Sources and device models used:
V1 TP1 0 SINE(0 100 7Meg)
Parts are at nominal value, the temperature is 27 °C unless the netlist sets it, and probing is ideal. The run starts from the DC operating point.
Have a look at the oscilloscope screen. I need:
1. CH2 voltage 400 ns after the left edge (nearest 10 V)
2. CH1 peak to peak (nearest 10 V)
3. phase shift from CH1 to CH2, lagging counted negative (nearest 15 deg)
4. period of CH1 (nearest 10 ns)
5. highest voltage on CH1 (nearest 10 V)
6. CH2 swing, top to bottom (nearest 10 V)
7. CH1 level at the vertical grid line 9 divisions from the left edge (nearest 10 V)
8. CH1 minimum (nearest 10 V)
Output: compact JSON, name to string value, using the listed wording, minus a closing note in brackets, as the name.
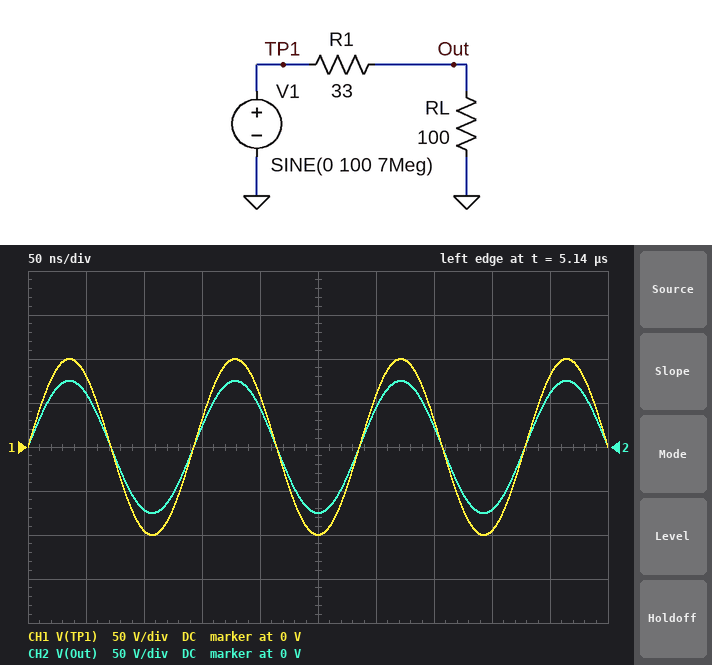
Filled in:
{"CH2 voltage 400 ns after the left edge": "-70 V", "CH1 peak to peak": "200 V", "phase shift from CH1 to CH2, lagging counted negative": "0 deg", "period of CH1": "140 ns", "highest voltage on CH1": "100 V", "CH2 swing, top to bottom": "150 V", "CH1 level at the vertical grid line 9 divisions from the left edge": "80 V", "CH1 minimum": "-100 V"}
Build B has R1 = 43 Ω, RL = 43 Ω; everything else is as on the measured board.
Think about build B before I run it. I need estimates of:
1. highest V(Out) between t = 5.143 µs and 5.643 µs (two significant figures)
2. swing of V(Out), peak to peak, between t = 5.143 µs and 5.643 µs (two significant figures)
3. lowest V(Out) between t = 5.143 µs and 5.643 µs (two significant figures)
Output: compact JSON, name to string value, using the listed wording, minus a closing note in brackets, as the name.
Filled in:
{"highest V(Out) between t = 5.143 µs and 5.643 µs": "50 V", "swing of V(Out), peak to peak, between t = 5.143 µs and 5.643 µs": "100 V", "lowest V(Out) between t = 5.143 µs and 5.643 µs": "-50 V"}
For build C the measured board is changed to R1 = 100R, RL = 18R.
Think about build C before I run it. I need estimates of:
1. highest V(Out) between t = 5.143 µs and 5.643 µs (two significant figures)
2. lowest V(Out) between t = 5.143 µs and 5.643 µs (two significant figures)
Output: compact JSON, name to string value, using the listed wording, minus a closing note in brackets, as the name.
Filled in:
{"highest V(Out) between t = 5.143 µs and 5.643 µs": "15 V", "lowest V(Out) between t = 5.143 µs and 5.643 µs": "-15 V"}
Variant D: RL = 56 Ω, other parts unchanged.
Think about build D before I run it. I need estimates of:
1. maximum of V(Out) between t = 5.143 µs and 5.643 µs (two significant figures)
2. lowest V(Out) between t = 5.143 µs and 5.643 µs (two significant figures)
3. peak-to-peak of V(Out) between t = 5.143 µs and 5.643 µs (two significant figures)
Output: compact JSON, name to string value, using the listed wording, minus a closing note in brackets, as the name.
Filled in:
{"maximum of V(Out) between t = 5.143 µs and 5.643 µs": "63 V", "lowest V(Out) between t = 5.143 µs and 5.643 µs": "-63 V", "peak-to-peak of V(Out) between t = 5.143 µs and 5.643 µs": "130 V"}
